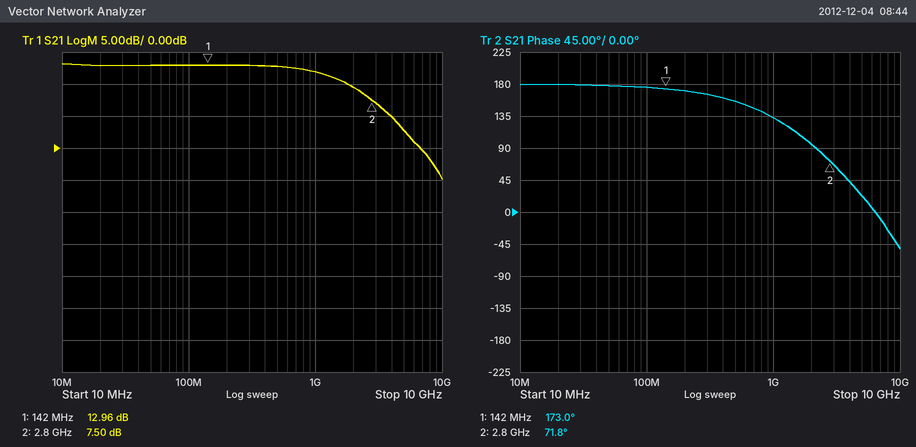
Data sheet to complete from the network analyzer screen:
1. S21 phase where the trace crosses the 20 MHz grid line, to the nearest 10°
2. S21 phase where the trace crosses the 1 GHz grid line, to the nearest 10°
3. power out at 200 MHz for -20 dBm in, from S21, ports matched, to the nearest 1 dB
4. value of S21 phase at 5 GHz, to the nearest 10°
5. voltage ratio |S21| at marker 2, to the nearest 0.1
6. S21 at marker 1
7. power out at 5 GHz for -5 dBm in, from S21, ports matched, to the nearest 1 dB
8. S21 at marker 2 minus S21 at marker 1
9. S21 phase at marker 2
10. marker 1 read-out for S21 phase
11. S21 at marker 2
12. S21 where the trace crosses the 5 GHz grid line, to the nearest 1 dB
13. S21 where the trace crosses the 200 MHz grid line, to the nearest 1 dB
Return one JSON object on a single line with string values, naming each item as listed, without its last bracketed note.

{"S21 phase where the trace crosses the 20 MHz grid line, to the nearest 10°": "180°", "S21 phase where the trace crosses the 1 GHz grid line, to the nearest 10°": "130°", "power out at 200 MHz for -20 dBm in, from S21, ports matched, to the nearest 1 dB": "-7 dBm", "value of S21 phase at 5 GHz, to the nearest 10°": "20°", "voltage ratio |S21| at marker 2, to the nearest 0.1": "2.4", "S21 at marker 1": "12.96 dB", "power out at 5 GHz for -5 dBm in, from S21, ports matched, to the nearest 1 dB": "-2 dBm", "S21 at marker 2 minus S21 at marker 1": "-5.46 dB", "S21 phase at marker 2": "71.8°", "marker 1 read-out for S21 phase": "173.0°", "S21 at marker 2": "7.50 dB", "S21 where the trace crosses the 5 GHz grid line, to the nearest 1 dB": "3 dB", "S21 where the trace crosses the 200 MHz grid line, to the nearest 1 dB": "13 dB"}
